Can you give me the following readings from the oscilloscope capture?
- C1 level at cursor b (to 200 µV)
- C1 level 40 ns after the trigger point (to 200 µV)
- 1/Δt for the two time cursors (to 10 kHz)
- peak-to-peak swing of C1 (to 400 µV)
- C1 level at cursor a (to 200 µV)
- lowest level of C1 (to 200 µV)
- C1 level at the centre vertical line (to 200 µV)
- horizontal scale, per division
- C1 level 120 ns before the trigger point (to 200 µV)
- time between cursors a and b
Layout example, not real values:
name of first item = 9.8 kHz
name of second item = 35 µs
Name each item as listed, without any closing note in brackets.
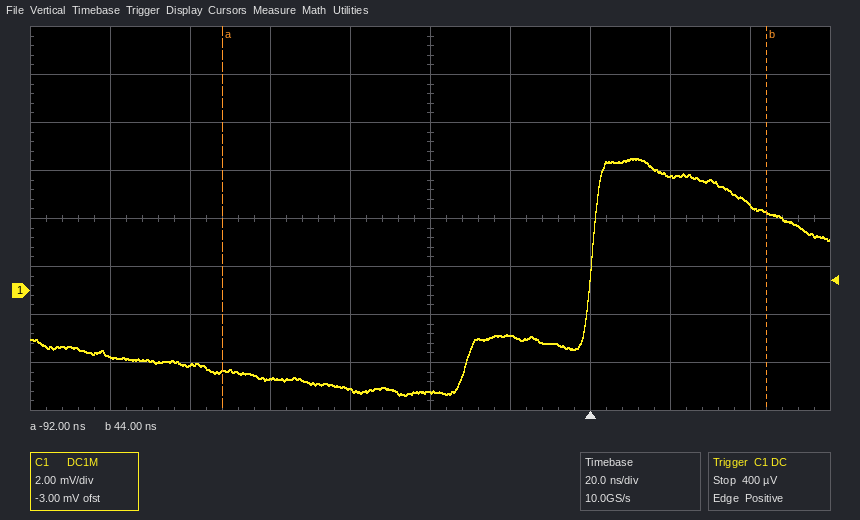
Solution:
C1 level at cursor b = 3.2 mV
C1 level 40 ns after the trigger point = 3.6 mV
1/Δt for the two time cursors = 7.35 MHz
peak-to-peak swing of C1 = 10.0 mV
C1 level at cursor a = -3.4 mV
lowest level of C1 = -4.4 mV
C1 level at the centre vertical line = -4.2 mV
horizontal scale, per division = 20 ns
C1 level 120 ns before the trigger point = -2.8 mV
time between cursors a and b = 136 ns
